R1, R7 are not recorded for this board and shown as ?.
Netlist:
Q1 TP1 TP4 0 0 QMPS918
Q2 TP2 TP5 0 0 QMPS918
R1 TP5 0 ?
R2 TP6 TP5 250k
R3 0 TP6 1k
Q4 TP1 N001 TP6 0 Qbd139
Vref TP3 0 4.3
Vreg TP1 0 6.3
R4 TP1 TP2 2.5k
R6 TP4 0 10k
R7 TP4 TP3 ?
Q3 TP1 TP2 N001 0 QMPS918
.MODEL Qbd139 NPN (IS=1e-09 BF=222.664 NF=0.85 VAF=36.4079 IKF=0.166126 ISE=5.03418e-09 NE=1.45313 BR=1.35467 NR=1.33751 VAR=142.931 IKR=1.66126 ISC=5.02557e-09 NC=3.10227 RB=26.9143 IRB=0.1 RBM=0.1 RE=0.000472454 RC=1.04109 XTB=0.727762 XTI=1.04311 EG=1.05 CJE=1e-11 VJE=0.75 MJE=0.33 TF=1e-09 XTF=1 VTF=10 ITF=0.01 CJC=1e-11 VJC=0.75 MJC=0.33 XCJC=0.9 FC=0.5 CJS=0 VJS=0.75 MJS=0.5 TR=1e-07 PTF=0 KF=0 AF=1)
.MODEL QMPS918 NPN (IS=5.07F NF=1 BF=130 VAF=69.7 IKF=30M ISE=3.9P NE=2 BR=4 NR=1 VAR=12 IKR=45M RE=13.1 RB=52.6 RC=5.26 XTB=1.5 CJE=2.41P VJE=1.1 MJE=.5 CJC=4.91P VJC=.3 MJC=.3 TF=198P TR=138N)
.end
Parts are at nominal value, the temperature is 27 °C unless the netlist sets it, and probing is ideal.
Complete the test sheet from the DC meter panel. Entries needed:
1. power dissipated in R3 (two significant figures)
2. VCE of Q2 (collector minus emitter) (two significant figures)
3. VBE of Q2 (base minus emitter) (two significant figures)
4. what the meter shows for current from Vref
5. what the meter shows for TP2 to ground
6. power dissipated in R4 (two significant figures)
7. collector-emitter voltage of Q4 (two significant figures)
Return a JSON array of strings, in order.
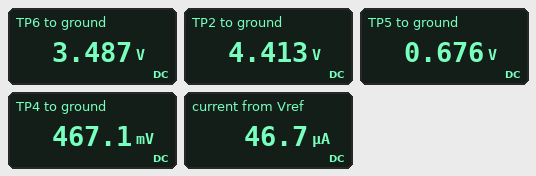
["12 mW", "4.4 V", "680 mV", "46.7 µA", "4.413 V", "1.4 mW", "2.8 V"]
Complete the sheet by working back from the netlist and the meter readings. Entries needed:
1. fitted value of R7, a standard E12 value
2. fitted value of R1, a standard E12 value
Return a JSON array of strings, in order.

["82 kΩ", "180 kΩ"]
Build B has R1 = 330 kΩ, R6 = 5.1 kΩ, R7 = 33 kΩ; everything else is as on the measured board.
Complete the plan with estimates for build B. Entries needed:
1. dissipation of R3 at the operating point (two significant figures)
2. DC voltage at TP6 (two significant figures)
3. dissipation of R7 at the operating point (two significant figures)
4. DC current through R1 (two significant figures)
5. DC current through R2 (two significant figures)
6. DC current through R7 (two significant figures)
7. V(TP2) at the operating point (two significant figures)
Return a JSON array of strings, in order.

["11 mW", "3.3 V", "420 µW", "2.1 µA", "10 µA", "110 µA", "4.2 V"]
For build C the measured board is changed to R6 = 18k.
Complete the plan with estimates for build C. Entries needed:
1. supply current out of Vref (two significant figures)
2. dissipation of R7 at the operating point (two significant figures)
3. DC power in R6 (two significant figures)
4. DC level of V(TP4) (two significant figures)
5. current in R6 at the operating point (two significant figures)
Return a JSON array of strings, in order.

["44 µA", "160 µW", "25 µW", "670 mV", "37 µA"]
